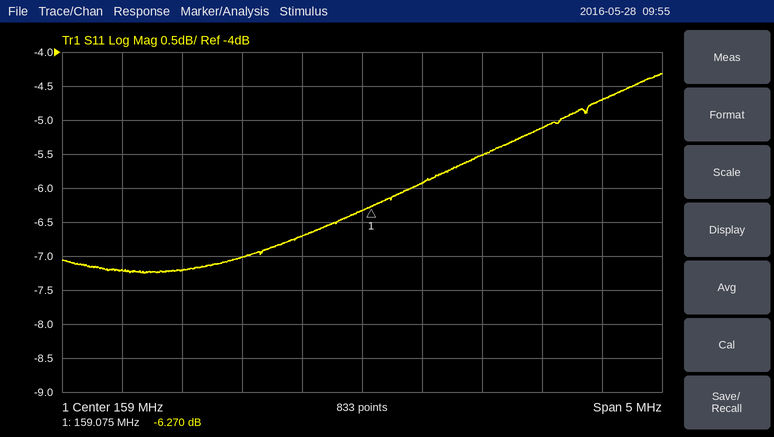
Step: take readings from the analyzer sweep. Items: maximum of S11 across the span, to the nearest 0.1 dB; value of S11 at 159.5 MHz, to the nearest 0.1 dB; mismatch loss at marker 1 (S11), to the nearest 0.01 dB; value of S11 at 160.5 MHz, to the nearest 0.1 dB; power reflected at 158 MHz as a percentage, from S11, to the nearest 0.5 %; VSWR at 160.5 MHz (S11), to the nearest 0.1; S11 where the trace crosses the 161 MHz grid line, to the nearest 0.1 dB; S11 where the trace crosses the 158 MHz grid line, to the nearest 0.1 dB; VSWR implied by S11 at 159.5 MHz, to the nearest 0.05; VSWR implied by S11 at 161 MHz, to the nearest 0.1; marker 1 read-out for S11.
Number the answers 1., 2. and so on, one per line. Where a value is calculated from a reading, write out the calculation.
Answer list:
1. -4.3 dB
2. -5.9 dB
3. −10 log10(1 − 10^(-6.27/10)) ≈ 1.17 dB
4. -5.1 dB
5. 10^(-7/10) ≈ 20.0 %
6. |Γ| = 10^(-5.1/20) = 0.5559; VSWR = (1 + 0.5559)/(1 − 0.5559) ≈ 3.5
7. -4.7 dB
8. -7.0 dB
9. |Γ| = 10^(-5.9/20) = 0.5070; VSWR = (1 + 0.5070)/(1 − 0.5070) ≈ 3.06, so 3.05 to the nearest 0.05
10. |Γ| = 10^(-4.7/20) = 0.5821; VSWR = (1 + 0.5821)/(1 − 0.5821) ≈ 3.8
11. -6.270 dB
